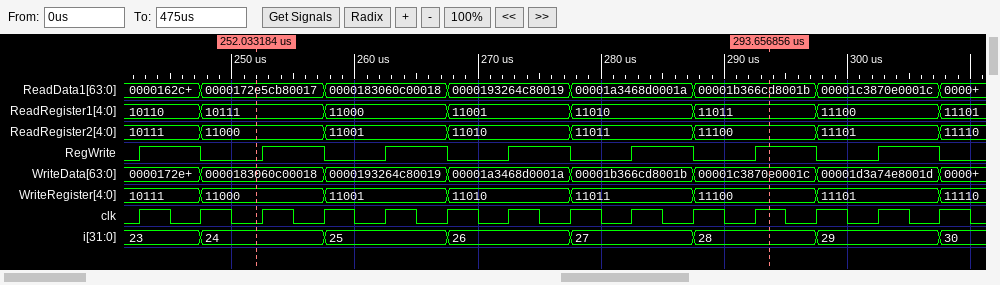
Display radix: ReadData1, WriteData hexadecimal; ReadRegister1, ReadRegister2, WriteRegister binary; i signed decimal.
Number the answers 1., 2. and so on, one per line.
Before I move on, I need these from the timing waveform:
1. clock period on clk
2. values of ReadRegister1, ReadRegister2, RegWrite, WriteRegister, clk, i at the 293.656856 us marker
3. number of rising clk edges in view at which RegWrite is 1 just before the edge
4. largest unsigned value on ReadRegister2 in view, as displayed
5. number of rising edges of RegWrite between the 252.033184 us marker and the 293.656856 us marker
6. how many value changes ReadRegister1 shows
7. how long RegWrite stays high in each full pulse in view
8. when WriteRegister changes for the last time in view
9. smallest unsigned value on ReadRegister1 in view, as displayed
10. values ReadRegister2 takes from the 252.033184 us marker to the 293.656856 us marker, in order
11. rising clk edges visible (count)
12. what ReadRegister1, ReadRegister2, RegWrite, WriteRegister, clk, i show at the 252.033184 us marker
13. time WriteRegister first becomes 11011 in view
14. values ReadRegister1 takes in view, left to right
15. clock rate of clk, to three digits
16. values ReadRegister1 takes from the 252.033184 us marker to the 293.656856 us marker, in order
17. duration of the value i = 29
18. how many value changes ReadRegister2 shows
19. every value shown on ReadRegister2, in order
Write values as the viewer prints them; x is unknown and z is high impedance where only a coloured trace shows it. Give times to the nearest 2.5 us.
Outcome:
1. 5 us
2. ReadRegister1=11011, ReadRegister2=11100, RegWrite=1, WriteRegister=11100, clk=1, i=28
3. 7
4. 11110
5. 5
6. 7
7. 5 us, 5 us, 5 us, 5 us, 5 us, 5 us, 5 us
8. 307.5 us
9. 10110
10. 11000, 11001, 11010, 11011, 11100
11. 14
12. ReadRegister1=10111, ReadRegister2=11000, RegWrite=0, WriteRegister=11000, clk=0, i=24
13. 277.5 us
14. 10110, 10111, 11000, 11001, 11010, 11011, 11100, 11101
15. 200 kHz
16. 10111, 11000, 11001, 11010, 11011
17. 10 us
18. 7
19. 10111, 11000, 11001, 11010, 11011, 11100, 11101, 11110
